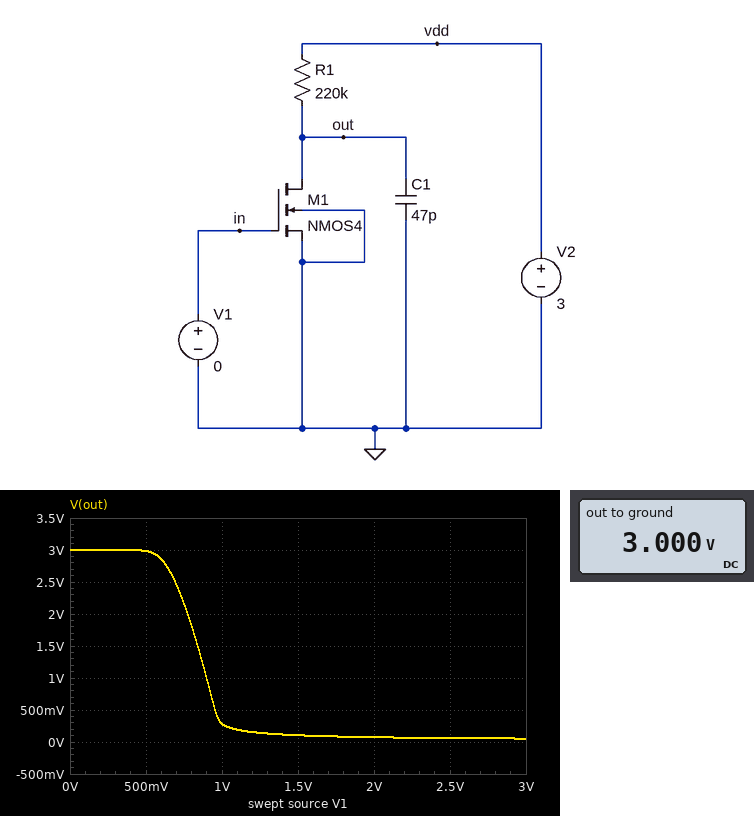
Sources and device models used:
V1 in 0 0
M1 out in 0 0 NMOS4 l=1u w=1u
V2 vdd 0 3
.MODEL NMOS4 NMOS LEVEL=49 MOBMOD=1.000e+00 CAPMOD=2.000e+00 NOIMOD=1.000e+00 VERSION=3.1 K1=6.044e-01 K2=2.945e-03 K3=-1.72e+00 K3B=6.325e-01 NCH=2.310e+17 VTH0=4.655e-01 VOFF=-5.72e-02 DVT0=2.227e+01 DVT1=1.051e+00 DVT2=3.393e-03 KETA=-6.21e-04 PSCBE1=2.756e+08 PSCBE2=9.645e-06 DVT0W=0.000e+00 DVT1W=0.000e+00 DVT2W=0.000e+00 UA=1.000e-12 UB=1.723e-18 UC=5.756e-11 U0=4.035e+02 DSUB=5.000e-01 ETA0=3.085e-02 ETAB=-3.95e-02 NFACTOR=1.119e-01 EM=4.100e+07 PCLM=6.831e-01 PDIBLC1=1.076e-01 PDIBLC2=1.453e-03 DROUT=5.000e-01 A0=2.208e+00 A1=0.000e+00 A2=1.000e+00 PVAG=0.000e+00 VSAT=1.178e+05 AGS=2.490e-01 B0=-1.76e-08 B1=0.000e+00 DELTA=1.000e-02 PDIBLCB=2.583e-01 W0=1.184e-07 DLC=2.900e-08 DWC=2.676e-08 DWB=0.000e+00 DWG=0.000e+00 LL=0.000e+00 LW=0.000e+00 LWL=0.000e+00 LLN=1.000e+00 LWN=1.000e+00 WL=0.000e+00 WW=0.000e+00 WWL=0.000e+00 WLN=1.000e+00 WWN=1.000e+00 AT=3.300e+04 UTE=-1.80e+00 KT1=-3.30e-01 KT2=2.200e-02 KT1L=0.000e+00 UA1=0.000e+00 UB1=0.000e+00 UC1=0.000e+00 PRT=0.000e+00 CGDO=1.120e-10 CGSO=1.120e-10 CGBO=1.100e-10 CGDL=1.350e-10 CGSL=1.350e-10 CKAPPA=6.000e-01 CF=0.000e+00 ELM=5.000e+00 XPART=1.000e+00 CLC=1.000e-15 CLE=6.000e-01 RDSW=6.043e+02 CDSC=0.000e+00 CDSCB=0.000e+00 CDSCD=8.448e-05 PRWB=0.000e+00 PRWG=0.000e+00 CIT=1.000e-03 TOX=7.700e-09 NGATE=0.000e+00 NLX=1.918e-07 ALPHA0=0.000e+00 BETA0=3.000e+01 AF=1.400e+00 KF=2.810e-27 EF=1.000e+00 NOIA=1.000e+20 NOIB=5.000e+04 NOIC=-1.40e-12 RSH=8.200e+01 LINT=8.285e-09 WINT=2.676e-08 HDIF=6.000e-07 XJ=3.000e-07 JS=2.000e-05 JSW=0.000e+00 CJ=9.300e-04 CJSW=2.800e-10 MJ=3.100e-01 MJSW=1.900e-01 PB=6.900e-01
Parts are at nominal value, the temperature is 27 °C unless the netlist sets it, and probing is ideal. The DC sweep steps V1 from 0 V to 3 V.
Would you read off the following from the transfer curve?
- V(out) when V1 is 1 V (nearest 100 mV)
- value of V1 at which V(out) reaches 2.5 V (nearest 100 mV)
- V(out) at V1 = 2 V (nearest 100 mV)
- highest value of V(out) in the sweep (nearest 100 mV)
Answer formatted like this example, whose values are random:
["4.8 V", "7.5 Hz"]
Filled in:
["300 mV", "700 mV", "100 mV", "3.0 V"]
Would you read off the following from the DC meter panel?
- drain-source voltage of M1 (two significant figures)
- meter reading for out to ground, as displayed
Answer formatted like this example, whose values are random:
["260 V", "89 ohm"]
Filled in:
["3.0 V", "3.000 V"]
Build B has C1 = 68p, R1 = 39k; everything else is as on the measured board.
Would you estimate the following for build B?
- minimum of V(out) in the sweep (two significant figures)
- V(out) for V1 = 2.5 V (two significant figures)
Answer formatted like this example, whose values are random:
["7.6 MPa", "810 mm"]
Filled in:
["300 mV", "350 mV"]
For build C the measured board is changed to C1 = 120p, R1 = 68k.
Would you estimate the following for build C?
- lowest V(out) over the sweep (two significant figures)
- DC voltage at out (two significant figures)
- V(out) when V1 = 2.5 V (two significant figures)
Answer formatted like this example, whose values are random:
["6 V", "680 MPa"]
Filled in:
["170 mV", "3.0 V", "200 mV"]
